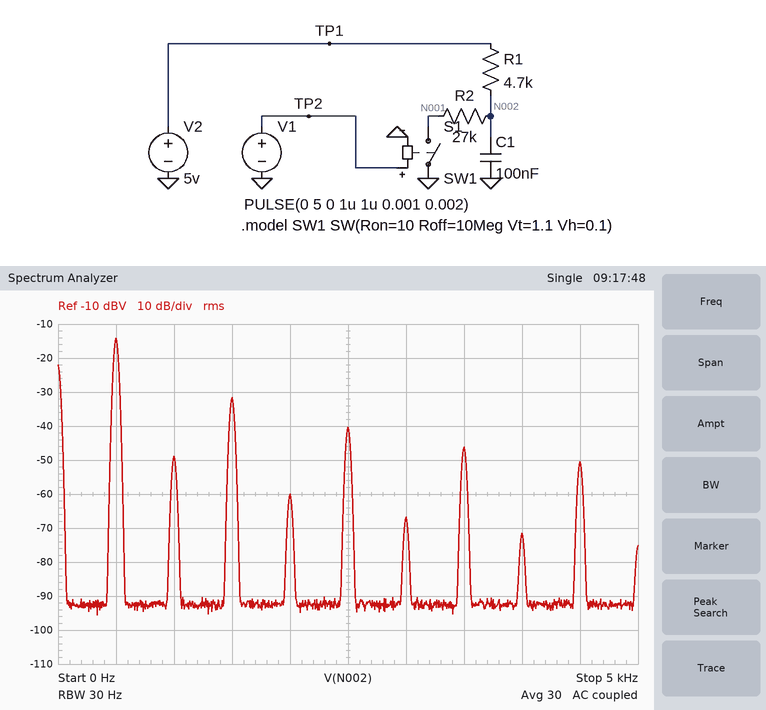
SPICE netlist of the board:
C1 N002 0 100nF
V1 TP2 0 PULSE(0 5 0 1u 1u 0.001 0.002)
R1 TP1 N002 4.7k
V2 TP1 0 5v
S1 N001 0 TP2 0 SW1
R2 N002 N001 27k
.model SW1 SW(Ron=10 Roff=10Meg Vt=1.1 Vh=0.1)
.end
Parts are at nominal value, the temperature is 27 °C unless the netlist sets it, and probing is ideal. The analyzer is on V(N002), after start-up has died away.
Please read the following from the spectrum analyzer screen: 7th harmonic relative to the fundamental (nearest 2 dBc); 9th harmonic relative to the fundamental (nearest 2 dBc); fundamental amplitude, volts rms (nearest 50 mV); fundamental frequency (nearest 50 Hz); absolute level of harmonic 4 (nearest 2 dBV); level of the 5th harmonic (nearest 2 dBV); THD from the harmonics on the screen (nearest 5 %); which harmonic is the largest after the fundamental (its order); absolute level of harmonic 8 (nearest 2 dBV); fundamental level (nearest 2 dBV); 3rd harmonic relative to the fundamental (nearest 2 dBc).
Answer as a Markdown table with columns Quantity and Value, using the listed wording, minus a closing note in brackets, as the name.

| Quantity | Value |
|---|---|
| 7th harmonic relative to the fundamental | -32 dBc |
| 9th harmonic relative to the fundamental | -36 dBc |
| fundamental amplitude, volts rms | 200 mV |
| fundamental frequency | 500 Hz |
| absolute level of harmonic 4 | -60 dBV |
| level of the 5th harmonic | -40 dBV |
| THD from the harmonics on the screen | 15 % |
| which harmonic is the largest after the fundamental | 3 |
| absolute level of harmonic 8 | -72 dBV |
| fundamental level | -14 dBV |
| 3rd harmonic relative to the fundamental | -18 dBc |
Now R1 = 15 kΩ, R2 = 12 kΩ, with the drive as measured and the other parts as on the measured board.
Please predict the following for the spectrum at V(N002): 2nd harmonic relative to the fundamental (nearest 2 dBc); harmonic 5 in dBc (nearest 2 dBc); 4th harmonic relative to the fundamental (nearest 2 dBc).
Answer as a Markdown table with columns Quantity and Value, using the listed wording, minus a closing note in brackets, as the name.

| Quantity | Value |
|---|---|
| 2nd harmonic relative to the fundamental | -26 dBc |
| harmonic 5 in dBc | -28 dBc |
| 4th harmonic relative to the fundamental | -38 dBc |
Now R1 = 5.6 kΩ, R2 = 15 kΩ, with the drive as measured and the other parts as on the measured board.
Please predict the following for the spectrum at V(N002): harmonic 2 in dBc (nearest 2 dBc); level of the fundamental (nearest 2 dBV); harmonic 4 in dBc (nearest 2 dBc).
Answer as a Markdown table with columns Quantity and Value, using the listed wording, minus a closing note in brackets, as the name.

| Quantity | Value |
|---|---|
| harmonic 2 in dBc | -30 dBc |
| level of the fundamental | -10 dBV |
| harmonic 4 in dBc | -40 dBc |
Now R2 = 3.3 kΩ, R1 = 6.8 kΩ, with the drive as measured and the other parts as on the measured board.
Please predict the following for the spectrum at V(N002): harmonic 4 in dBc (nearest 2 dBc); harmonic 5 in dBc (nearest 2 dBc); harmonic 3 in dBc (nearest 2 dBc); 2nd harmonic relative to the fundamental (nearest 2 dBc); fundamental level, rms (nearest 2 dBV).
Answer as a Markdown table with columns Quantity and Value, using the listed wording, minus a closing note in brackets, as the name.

| Quantity | Value |
|---|---|
| harmonic 4 in dBc | -28 dBc |
| harmonic 5 in dBc | -24 dBc |
| harmonic 3 in dBc | -16 dBc |
| 2nd harmonic relative to the fundamental | -18 dBc |
| fundamental level, rms | -2 dBV |
